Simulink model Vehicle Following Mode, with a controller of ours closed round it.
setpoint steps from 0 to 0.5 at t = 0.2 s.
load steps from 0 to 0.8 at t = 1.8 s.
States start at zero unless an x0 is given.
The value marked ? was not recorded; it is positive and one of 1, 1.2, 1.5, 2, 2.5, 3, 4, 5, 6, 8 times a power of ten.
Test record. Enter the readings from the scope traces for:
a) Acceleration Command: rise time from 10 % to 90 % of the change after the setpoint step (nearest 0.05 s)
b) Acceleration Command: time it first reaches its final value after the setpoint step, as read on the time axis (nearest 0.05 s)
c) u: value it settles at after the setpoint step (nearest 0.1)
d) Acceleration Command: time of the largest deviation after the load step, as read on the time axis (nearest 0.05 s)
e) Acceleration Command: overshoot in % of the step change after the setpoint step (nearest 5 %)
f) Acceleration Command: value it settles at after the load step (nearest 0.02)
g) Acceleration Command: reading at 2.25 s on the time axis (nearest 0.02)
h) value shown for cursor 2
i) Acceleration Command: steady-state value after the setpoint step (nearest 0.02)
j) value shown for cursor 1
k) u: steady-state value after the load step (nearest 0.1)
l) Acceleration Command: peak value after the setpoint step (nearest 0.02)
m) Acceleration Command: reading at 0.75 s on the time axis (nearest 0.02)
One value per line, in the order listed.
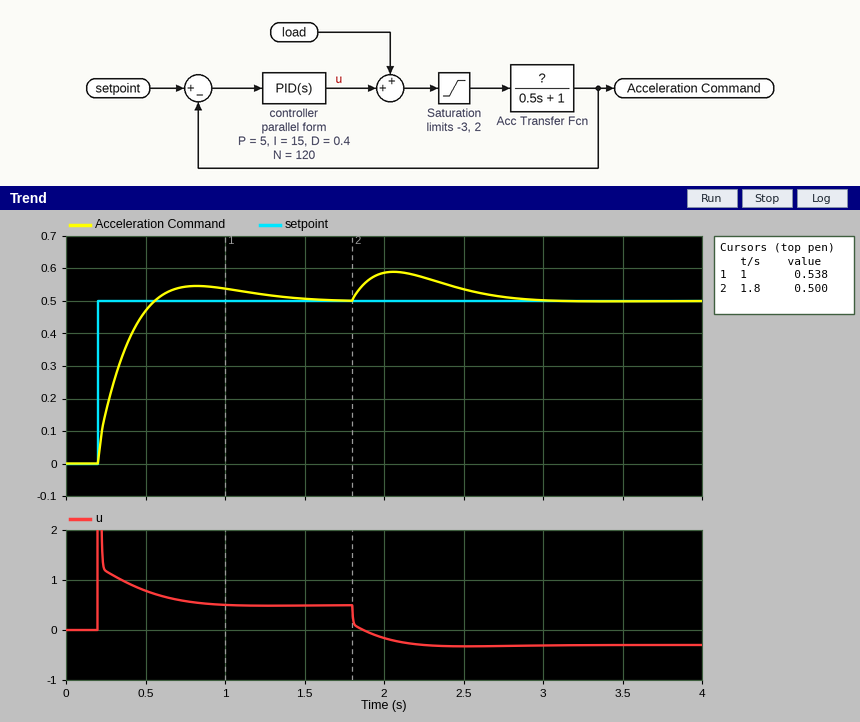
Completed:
0.25 s
0.55 s
0.5
2.05 s
10 %
0.50
0.58
0.500
0.50
0.538
-0.3
0.54
0.54
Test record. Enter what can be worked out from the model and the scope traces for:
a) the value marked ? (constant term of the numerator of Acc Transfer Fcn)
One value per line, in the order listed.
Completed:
1
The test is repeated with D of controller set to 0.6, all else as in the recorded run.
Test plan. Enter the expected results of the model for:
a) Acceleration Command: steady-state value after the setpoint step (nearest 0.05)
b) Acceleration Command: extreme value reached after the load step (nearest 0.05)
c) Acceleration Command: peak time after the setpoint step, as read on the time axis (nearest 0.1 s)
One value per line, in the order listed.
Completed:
0.50
0.60
0.9 s
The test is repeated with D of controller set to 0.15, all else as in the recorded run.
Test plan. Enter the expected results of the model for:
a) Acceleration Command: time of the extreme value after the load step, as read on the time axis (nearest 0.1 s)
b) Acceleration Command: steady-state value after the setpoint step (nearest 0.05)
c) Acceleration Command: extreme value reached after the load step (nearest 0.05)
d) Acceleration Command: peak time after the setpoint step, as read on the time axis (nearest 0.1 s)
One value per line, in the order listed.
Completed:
2.0 s
0.50
0.60
0.7 s
